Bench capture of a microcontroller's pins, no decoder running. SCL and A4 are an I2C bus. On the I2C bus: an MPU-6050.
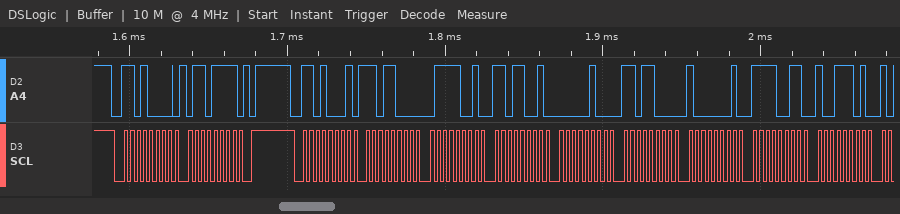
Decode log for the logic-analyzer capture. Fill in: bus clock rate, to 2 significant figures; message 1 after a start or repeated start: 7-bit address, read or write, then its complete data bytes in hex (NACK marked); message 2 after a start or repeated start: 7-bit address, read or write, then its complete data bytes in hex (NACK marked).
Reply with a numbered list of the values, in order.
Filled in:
1. 250 kHz
2. 0x68 write: 6F
3. 0x68 read: D8 79 D9 04 D8 81 F3 9D
